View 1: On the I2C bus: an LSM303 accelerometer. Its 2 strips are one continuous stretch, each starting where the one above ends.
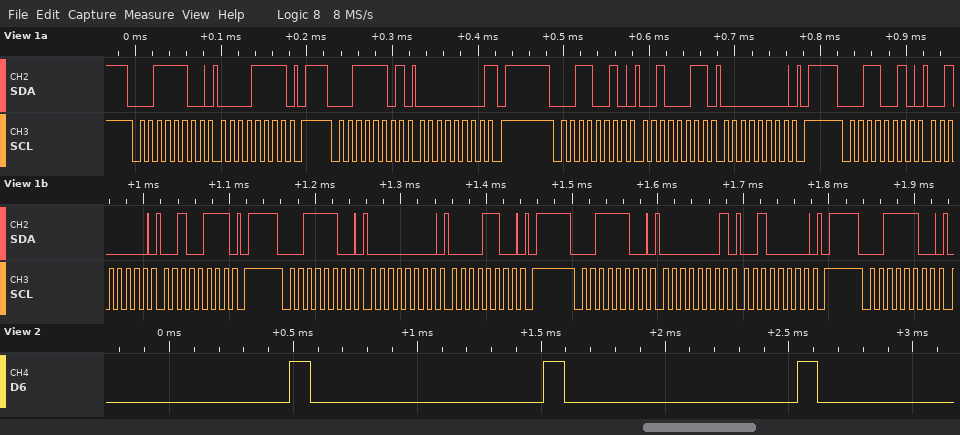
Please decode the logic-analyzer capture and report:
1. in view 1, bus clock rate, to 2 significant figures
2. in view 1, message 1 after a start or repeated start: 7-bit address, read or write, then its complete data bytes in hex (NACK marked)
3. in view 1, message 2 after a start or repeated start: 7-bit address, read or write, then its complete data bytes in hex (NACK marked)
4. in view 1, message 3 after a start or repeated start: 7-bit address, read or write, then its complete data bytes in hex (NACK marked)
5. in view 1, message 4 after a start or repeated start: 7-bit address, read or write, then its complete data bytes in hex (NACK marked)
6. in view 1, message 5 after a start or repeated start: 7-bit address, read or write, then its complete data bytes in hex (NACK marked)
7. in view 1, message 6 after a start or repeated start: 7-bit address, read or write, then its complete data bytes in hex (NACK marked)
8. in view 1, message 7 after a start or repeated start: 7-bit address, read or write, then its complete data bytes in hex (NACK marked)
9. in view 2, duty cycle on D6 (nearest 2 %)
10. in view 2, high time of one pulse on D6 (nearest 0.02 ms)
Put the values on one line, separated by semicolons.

100 kHz; 0x1E write: 0F; 0x1E read: 00 NACK; 0x19 write: 23 00; 0x19 write: 20 27; 0x1E write: 00 0C; 0x1E write: 01 20; 0x1E write; 8 %; 0.08 ms
